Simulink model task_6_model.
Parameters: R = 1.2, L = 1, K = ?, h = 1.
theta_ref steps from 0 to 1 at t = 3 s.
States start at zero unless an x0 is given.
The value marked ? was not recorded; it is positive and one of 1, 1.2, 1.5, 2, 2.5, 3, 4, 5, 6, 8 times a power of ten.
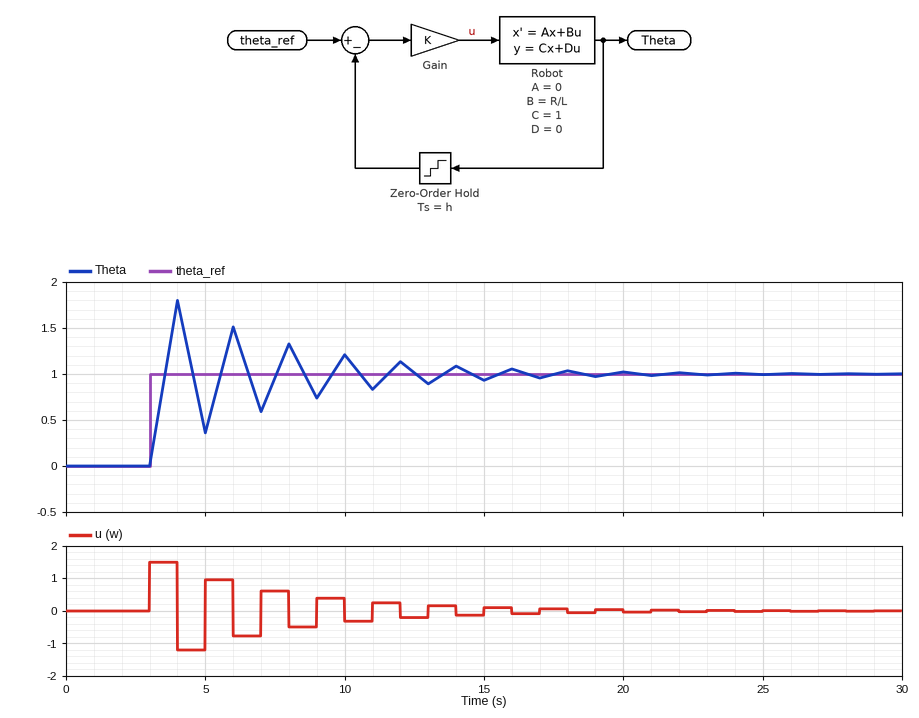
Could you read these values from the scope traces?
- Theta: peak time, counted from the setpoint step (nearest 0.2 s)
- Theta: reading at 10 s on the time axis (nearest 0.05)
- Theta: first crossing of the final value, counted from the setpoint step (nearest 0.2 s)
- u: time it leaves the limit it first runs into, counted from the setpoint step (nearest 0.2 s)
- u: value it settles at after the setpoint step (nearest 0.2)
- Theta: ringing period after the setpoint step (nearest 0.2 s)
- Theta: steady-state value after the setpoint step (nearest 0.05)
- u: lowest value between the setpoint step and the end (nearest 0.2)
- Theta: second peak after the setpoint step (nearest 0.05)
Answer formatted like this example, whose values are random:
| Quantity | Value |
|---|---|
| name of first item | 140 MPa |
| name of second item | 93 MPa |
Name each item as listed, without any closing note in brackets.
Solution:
| Quantity | Value |
|---|---|
| Theta: peak time, counted from the setpoint step | 1.0 s |
| Theta: reading at 10 s on the time axis | 1.20 |
| Theta: first crossing of the final value, counted from the setpoint step | 0.6 s |
| u: time it leaves the limit it first runs into, counted from the setpoint step | 1.0 s |
| u: value it settles at after the setpoint step | 0.0 |
| Theta: ringing period after the setpoint step | 2.0 s |
| Theta: steady-state value after the setpoint step | 1.00 |
| u: lowest value between the setpoint step and the end | -1.2 |
| Theta: second peak after the setpoint step | 1.50 |
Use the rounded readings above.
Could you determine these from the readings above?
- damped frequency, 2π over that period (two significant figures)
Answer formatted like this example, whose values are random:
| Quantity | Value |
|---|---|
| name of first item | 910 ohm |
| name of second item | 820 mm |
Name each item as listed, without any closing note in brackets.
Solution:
| Quantity | Value |
|---|---|
| damped frequency, 2π over that period | 3.1 rad/s |
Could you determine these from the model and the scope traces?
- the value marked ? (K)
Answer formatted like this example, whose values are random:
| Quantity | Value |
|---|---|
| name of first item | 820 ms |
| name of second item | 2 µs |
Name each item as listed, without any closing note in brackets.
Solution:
| Quantity | Value |
|---|---|
| the value marked ? | 1.5 |
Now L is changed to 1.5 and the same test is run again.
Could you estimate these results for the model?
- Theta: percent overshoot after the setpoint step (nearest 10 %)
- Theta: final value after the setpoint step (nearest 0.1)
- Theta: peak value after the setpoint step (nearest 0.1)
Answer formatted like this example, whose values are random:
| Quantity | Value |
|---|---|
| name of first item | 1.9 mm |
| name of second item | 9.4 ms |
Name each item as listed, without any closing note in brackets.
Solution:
| Quantity | Value |
|---|---|
| Theta: percent overshoot after the setpoint step | 20 % |
| Theta: final value after the setpoint step | 1.0 |
| Theta: peak value after the setpoint step | 1.2 |
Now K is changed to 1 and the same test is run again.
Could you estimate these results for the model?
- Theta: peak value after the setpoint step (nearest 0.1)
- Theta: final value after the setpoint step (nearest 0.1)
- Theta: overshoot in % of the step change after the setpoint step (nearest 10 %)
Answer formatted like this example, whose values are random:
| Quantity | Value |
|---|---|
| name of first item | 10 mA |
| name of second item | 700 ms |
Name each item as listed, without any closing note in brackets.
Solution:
| Quantity | Value |
|---|---|
| Theta: peak value after the setpoint step | 1.2 |
| Theta: final value after the setpoint step | 1.0 |
| Theta: overshoot in % of the step change after the setpoint step | 20 % |
